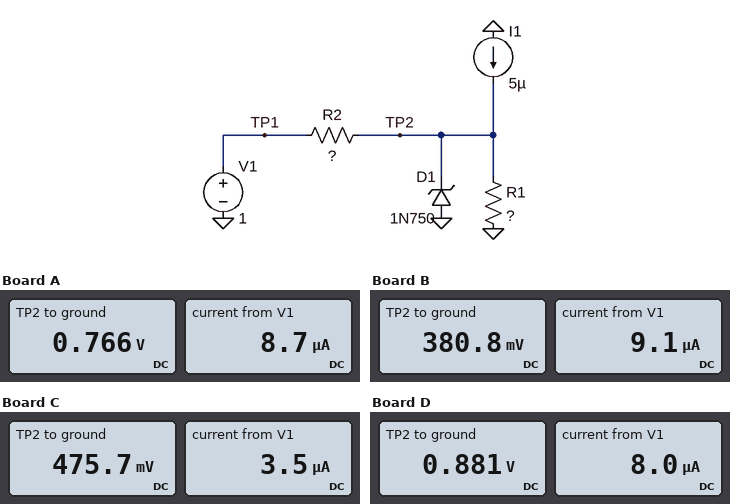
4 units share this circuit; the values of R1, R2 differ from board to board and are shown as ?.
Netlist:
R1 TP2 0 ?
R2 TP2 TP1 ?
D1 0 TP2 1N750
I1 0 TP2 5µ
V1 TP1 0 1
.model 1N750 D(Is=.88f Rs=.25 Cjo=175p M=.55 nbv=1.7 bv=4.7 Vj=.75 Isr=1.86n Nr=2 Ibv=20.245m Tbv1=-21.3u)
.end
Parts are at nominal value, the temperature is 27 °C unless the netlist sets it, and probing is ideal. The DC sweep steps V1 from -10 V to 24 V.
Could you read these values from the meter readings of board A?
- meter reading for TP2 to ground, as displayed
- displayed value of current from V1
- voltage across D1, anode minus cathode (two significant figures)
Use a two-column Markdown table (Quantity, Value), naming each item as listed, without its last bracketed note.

| Quantity | Value |
|---|---|
| meter reading for TP2 to ground, as displayed | 0.766 V |
| displayed value of current from V1 | 8.7 µA |
| voltage across D1, anode minus cathode | -770 mV |
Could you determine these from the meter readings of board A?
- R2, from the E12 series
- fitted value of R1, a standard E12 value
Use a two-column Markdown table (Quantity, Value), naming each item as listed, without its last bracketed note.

| Quantity | Value |
|---|---|
| R2, from the E12 series | 27 kΩ |
| fitted value of R1, a standard E12 value | 56 kΩ |
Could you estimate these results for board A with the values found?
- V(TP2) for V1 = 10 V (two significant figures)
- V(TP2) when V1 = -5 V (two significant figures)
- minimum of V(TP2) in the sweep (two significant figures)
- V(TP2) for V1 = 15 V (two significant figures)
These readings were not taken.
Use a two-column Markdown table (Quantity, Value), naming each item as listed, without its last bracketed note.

| Quantity | Value |
|---|---|
| V(TP2) for V1 = 10 V | 4.5 V |
| V(TP2) when V1 = -5 V | -620 mV |
| minimum of V(TP2) in the sweep | -660 mV |
| V(TP2) for V1 = 15 V | 4.5 V |
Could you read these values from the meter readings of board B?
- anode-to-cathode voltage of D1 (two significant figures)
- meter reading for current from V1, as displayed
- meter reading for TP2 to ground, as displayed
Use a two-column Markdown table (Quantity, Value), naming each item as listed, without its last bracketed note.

| Quantity | Value |
|---|---|
| anode-to-cathode voltage of D1 | -380 mV |
| meter reading for current from V1, as displayed | 9.1 µA |
| meter reading for TP2 to ground, as displayed | 380.8 mV |
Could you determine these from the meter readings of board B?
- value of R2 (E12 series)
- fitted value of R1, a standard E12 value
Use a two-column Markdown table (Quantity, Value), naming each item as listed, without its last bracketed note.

| Quantity | Value |
|---|---|
| value of R2 | 68 kΩ |
| fitted value of R1, a standard E12 value | 27 kΩ |
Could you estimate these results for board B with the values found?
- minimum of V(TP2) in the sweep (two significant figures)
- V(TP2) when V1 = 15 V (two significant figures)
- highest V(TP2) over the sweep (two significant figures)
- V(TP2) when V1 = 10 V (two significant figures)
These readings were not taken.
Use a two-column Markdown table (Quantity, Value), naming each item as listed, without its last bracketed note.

| Quantity | Value |
|---|---|
| minimum of V(TP2) in the sweep | -610 mV |
| V(TP2) when V1 = 15 V | 4.3 V |
| highest V(TP2) over the sweep | 4.5 V |
| V(TP2) when V1 = 10 V | 2.9 V |
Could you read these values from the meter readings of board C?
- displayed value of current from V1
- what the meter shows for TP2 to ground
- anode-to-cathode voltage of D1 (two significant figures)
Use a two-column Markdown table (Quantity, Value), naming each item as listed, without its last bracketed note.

| Quantity | Value |
|---|---|
| displayed value of current from V1 | 3.5 µA |
| what the meter shows for TP2 to ground | 475.7 mV |
| anode-to-cathode voltage of D1 | -480 mV |
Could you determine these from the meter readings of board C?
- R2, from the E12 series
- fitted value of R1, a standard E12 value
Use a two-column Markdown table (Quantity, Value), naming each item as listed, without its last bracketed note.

| Quantity | Value |
|---|---|
| R2, from the E12 series | 150 kΩ |
| fitted value of R1, a standard E12 value | 56 kΩ |
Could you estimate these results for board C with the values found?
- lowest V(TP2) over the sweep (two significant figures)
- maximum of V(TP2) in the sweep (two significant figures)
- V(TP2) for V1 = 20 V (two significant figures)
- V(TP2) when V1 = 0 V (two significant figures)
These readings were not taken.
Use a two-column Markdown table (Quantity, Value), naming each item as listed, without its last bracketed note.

| Quantity | Value |
|---|---|
| lowest V(TP2) over the sweep | -560 mV |
| maximum of V(TP2) in the sweep | 4.4 V |
| V(TP2) for V1 = 20 V | 4.4 V |
| V(TP2) when V1 = 0 V | 200 mV |
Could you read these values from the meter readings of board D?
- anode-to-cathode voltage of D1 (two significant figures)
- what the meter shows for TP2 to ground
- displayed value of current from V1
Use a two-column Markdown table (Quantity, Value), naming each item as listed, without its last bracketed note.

| Quantity | Value |
|---|---|
| anode-to-cathode voltage of D1 | -880 mV |
| what the meter shows for TP2 to ground | 0.881 V |
| displayed value of current from V1 | 8.0 µA |
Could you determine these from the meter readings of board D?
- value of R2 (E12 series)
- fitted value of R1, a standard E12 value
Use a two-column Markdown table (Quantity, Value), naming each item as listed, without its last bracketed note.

| Quantity | Value |
|---|---|
| value of R2 | 15 kΩ |
| fitted value of R1, a standard E12 value | 68 kΩ |
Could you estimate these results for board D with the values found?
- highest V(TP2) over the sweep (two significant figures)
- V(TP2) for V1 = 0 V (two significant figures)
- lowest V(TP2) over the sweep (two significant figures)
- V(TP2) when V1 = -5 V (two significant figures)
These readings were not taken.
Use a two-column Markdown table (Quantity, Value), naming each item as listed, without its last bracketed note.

| Quantity | Value |
|---|---|
| highest V(TP2) over the sweep | 4.6 V |
| V(TP2) for V1 = 0 V | 61 mV |
| lowest V(TP2) over the sweep | -690 mV |
| V(TP2) when V1 = -5 V | -650 mV |
